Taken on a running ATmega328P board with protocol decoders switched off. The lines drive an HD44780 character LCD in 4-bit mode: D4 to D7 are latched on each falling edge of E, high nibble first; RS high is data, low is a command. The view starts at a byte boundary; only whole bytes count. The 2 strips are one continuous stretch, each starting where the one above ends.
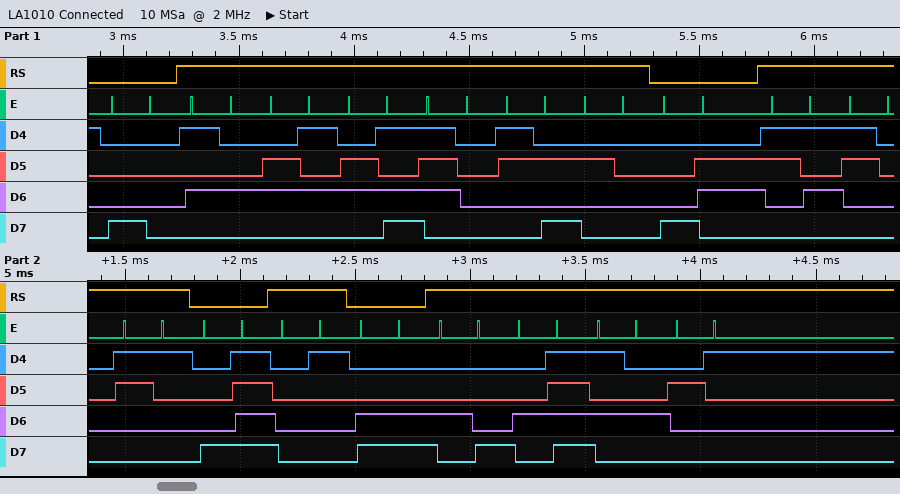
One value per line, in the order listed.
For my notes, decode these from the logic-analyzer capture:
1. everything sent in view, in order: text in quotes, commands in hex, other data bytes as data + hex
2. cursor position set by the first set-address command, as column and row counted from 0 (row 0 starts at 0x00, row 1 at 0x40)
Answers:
0x80 "Temp: " 0x86 "501" 0x8F data 01 0xCC "HOT!"
column 0, row 0
